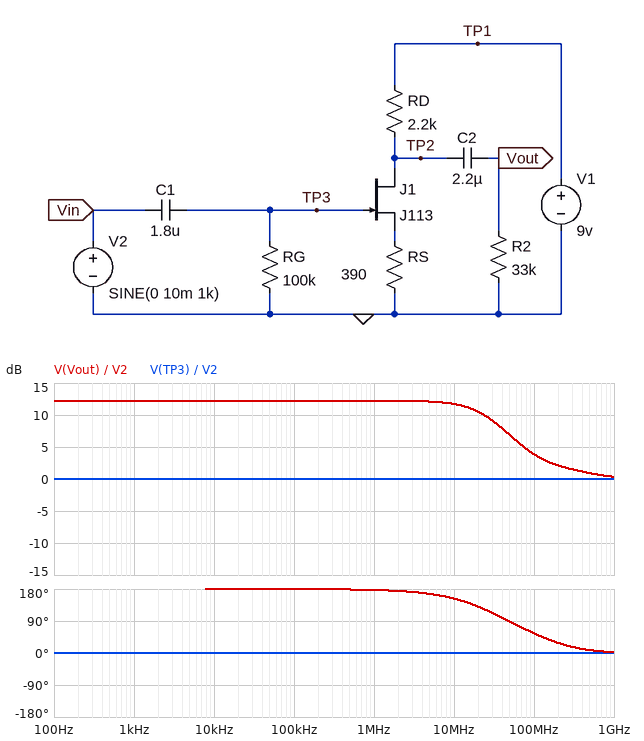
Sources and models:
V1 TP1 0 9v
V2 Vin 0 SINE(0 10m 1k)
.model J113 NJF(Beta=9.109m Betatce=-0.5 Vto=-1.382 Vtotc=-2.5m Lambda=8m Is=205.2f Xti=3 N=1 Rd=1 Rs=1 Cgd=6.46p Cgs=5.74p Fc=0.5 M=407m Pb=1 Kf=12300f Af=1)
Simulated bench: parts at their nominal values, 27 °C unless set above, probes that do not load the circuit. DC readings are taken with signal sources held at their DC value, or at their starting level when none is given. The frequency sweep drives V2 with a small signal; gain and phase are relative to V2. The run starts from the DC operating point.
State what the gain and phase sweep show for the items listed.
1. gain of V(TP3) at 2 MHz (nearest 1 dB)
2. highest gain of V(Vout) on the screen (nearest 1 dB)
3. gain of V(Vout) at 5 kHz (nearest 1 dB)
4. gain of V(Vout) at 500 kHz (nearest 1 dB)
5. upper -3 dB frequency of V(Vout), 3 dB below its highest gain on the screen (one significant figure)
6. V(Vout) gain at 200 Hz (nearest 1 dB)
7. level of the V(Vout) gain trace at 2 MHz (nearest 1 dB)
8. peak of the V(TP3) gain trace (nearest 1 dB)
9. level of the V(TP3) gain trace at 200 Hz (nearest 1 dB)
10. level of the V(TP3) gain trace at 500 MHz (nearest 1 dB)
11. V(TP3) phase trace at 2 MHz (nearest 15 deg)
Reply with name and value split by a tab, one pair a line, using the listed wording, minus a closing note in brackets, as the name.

gain of V(TP3) at 2 MHz	0 dB
highest gain of V(Vout) on the screen	12 dB
gain of V(Vout) at 5 kHz	12 dB
gain of V(Vout) at 500 kHz	12 dB
upper -3 dB frequency of V(Vout), 3 dB below its highest gain on the screen	30 MHz
V(Vout) gain at 200 Hz	12 dB
level of the V(Vout) gain trace at 2 MHz	12 dB
peak of the V(TP3) gain trace	0 dB
level of the V(TP3) gain trace at 200 Hz	0 dB
level of the V(TP3) gain trace at 500 MHz	0 dB
V(TP3) phase trace at 2 MHz	0 deg
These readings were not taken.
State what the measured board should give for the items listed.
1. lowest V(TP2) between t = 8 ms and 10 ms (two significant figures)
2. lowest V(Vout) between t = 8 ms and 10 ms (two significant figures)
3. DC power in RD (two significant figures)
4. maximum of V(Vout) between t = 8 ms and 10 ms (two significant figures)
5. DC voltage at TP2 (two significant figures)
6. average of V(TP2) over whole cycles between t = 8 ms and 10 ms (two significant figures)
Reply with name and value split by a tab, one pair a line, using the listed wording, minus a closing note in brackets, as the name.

lowest V(TP2) between t = 8 ms and 10 ms	4.0 V
lowest V(Vout) between t = 8 ms and 10 ms	-41 mV
DC power in RD	11 mW
maximum of V(Vout) between t = 8 ms and 10 ms	41 mV
DC voltage at TP2	4.0 V
average of V(TP2) over whole cycles between t = 8 ms and 10 ms	4.0 V
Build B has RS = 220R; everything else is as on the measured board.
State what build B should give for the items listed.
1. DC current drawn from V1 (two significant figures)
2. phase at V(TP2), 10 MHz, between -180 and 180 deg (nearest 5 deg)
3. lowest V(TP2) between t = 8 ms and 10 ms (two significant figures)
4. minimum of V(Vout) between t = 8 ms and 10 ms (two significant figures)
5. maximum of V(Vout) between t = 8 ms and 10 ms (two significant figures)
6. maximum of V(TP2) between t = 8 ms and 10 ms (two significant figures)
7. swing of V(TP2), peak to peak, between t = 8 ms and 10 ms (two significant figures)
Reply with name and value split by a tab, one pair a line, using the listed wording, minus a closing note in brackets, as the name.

DC current drawn from V1	3.5 mA
phase at V(TP2), 10 MHz, between -180 and 180 deg	150 deg
lowest V(TP2) between t = 8 ms and 10 ms	1.3 V
minimum of V(Vout) between t = 8 ms and 10 ms	-43 mV
maximum of V(Vout) between t = 8 ms and 10 ms	64 mV
maximum of V(TP2) between t = 8 ms and 10 ms	1.4 V
swing of V(TP2), peak to peak, between t = 8 ms and 10 ms	110 mV
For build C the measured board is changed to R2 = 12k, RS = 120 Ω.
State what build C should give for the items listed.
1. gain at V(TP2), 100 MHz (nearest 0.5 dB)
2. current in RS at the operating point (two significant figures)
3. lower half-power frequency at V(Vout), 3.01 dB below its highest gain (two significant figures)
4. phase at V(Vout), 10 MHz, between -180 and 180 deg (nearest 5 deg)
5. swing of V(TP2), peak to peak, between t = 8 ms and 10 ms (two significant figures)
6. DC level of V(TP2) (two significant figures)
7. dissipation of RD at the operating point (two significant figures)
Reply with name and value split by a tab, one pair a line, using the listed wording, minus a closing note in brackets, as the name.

gain at V(TP2), 100 MHz	-2.0 dB
current in RS at the operating point	3.8 mA
lower half-power frequency at V(Vout), 3.01 dB below its highest gain	90 MHz
phase at V(Vout), 10 MHz, between -180 and 180 deg	160 deg
swing of V(TP2), peak to peak, between t = 8 ms and 10 ms	6.8 mV
DC level of V(TP2)	720 mV
dissipation of RD at the operating point	31 mW
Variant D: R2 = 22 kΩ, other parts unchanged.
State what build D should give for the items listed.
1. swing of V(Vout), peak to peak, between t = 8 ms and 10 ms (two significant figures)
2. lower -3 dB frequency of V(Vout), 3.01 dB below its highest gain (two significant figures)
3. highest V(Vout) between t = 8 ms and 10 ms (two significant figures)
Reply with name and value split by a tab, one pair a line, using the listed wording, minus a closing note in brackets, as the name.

swing of V(Vout), peak to peak, between t = 8 ms and 10 ms	79 mV
lower -3 dB frequency of V(Vout), 3.01 dB below its highest gain	3.2 Hz
highest V(Vout) between t = 8 ms and 10 ms	40 mV
